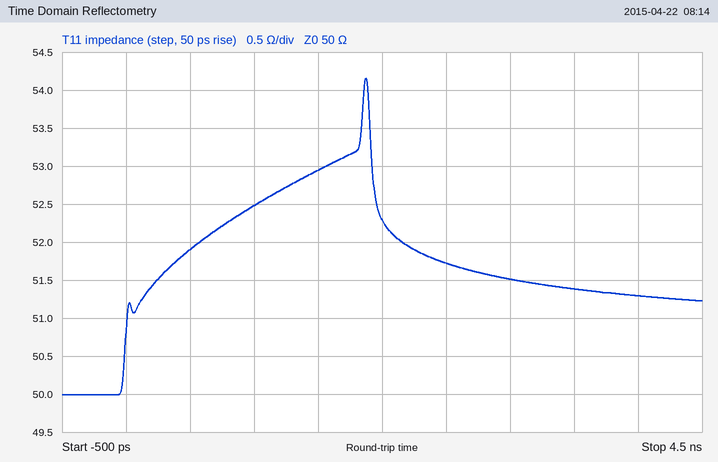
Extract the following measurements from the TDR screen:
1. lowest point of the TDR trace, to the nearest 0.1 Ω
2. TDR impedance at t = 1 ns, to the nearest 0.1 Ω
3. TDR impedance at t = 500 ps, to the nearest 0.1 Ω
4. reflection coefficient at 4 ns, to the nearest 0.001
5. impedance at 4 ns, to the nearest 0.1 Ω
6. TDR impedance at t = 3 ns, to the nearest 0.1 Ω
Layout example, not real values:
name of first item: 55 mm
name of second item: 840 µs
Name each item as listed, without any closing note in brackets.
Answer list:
lowest point of the TDR trace, to the nearest 0.1 Ω: 50.0 Ω
TDR impedance at t = 1 ns, to the nearest 0.1 Ω: 52.5 Ω
TDR impedance at t = 500 ps, to the nearest 0.1 Ω: 51.9 Ω
reflection coefficient at 4 ns, to the nearest 0.001: +0.013
impedance at 4 ns, to the nearest 0.1 Ω: 51.3 Ω
TDR impedance at t = 3 ns, to the nearest 0.1 Ω: 51.5 Ω
